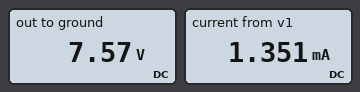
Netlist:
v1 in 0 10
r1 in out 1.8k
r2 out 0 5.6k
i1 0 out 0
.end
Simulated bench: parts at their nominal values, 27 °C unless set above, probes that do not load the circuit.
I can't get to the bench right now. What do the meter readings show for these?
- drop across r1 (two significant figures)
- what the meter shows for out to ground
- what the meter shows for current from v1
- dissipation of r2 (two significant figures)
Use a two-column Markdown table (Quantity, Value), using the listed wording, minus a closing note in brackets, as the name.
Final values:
| Quantity | Value |
|---|---|
| drop across r1 | 2.4 V |
| what the meter shows for out to ground | 7.57 V |
| what the meter shows for current from v1 | 1.351 mA |
| dissipation of r2 | 10 mW |
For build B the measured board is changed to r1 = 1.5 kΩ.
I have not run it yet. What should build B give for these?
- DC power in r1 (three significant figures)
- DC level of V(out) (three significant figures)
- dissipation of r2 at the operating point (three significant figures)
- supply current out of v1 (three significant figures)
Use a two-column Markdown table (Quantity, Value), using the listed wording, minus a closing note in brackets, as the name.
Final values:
| Quantity | Value |
|---|---|
| DC power in r1 | 2.98 mW |
| DC level of V(out) | 7.89 V |
| dissipation of r2 at the operating point | 11.1 mW |
| supply current out of v1 | 1.41 mA |
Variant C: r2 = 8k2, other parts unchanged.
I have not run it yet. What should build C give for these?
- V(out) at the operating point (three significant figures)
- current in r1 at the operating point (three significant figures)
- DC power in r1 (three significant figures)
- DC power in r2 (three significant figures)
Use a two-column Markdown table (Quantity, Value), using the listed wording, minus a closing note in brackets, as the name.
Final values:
| Quantity | Value |
|---|---|
| V(out) at the operating point | 8.20 V |
| current in r1 at the operating point | 1.00 mA |
| DC power in r1 | 1.80 mW |
| DC power in r2 | 8.20 mW |
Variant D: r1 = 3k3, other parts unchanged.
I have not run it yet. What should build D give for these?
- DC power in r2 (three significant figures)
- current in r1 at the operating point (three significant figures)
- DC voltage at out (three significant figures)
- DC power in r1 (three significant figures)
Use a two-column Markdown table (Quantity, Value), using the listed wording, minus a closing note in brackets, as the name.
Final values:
| Quantity | Value |
|---|---|
| DC power in r2 | 7.07 mW |
| current in r1 at the operating point | 1.12 mA |
| DC voltage at out | 6.29 V |
| DC power in r1 | 4.17 mW |
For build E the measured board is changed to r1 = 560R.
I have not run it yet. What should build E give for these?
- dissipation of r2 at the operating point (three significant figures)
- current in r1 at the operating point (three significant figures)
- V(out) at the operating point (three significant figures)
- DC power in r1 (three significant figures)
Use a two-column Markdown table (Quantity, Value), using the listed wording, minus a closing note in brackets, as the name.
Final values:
| Quantity | Value |
|---|---|
| dissipation of r2 at the operating point | 14.8 mW |
| current in r1 at the operating point | 1.62 mA |
| V(out) at the operating point | 9.09 V |
| DC power in r1 | 1.48 mW |
